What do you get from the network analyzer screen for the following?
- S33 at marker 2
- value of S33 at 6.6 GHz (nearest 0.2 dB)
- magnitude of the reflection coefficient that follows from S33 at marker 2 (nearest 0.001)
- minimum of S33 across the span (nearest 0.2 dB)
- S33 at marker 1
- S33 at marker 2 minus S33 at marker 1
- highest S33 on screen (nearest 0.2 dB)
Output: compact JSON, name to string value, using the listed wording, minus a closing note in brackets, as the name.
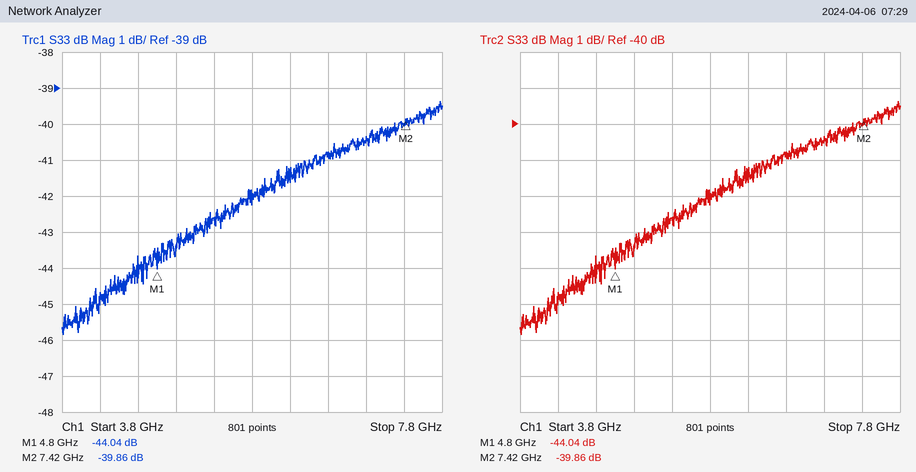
{"S33 at marker 2": "-39.86 dB", "value of S33 at 6.6 GHz": "-40.8 dB", "magnitude of the reflection coefficient that follows from S33 at marker 2": "0.010", "minimum of S33 across the span": "-45.8 dB", "S33 at marker 1": "-44.04 dB", "S33 at marker 2 minus S33 at marker 1": "4.18 dB", "highest S33 on screen": "-39.4 dB"}
